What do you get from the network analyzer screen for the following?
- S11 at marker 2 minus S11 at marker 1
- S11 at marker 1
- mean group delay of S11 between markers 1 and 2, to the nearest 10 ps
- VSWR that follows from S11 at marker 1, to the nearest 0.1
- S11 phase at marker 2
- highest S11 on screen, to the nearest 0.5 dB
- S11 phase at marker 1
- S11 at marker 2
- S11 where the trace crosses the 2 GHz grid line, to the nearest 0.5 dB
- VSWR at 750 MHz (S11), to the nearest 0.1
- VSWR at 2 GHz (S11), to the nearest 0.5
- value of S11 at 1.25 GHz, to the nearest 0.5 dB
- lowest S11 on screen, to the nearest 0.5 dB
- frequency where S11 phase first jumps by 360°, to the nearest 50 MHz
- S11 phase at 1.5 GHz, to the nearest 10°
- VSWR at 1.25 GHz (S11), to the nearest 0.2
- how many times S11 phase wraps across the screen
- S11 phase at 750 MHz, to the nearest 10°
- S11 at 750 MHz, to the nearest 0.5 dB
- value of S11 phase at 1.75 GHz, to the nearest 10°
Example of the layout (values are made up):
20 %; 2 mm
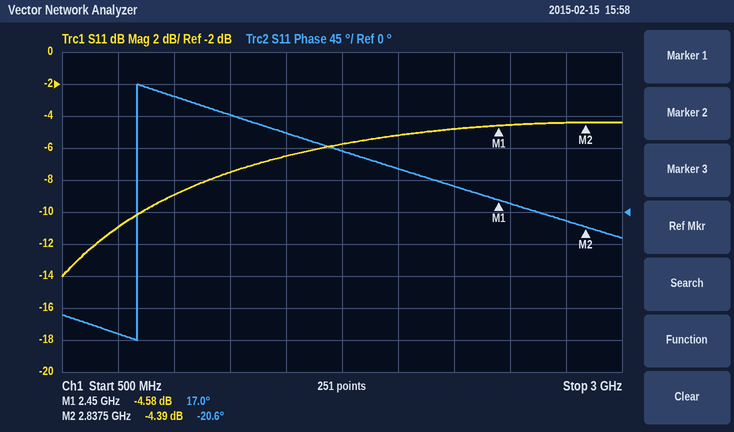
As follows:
0.19 dB; -4.58 dB; 270 ps; 3.9; -20.6°; -4.5 dB; 17.0°; -4.39 dB; -5.0 dB; 1.8; 3.5; -7.5 dB; -14.0 dB; 850 MHz; 110°; 2.4; 1; -170°; -11.0 dB; 90°
